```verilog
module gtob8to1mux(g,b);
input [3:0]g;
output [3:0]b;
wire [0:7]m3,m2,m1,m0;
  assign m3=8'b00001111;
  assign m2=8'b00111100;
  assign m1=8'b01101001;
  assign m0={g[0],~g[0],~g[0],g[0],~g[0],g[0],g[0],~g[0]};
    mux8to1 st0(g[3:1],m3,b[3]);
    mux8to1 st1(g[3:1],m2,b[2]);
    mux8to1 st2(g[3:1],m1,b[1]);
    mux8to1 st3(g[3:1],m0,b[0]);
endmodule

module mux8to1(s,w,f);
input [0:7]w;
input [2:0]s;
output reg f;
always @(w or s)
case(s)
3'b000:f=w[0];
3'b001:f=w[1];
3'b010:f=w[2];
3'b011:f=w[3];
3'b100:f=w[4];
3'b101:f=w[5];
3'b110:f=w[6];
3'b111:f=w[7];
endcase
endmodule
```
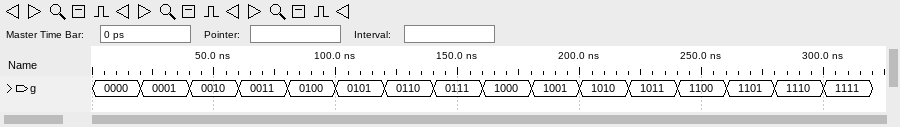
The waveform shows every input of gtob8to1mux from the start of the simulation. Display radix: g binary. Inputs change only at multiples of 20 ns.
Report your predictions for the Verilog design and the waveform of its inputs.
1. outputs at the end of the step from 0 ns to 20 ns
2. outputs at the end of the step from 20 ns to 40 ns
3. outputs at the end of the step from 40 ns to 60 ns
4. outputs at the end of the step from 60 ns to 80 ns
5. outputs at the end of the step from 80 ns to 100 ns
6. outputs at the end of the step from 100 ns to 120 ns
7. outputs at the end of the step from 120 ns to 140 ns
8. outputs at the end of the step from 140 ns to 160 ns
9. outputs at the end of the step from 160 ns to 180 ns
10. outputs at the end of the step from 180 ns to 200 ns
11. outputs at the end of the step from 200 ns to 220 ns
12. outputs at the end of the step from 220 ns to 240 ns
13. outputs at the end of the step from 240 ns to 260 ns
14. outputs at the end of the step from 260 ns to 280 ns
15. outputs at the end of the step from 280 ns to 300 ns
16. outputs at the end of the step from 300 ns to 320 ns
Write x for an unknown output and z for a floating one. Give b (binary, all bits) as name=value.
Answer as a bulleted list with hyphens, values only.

- b=0000
- b=0001
- b=0011
- b=0010
- b=0111
- b=0110
- b=0100
- b=0101
- b=1111
- b=1110
- b=1100
- b=1101
- b=1000
- b=1001
- b=1011
- b=1010
